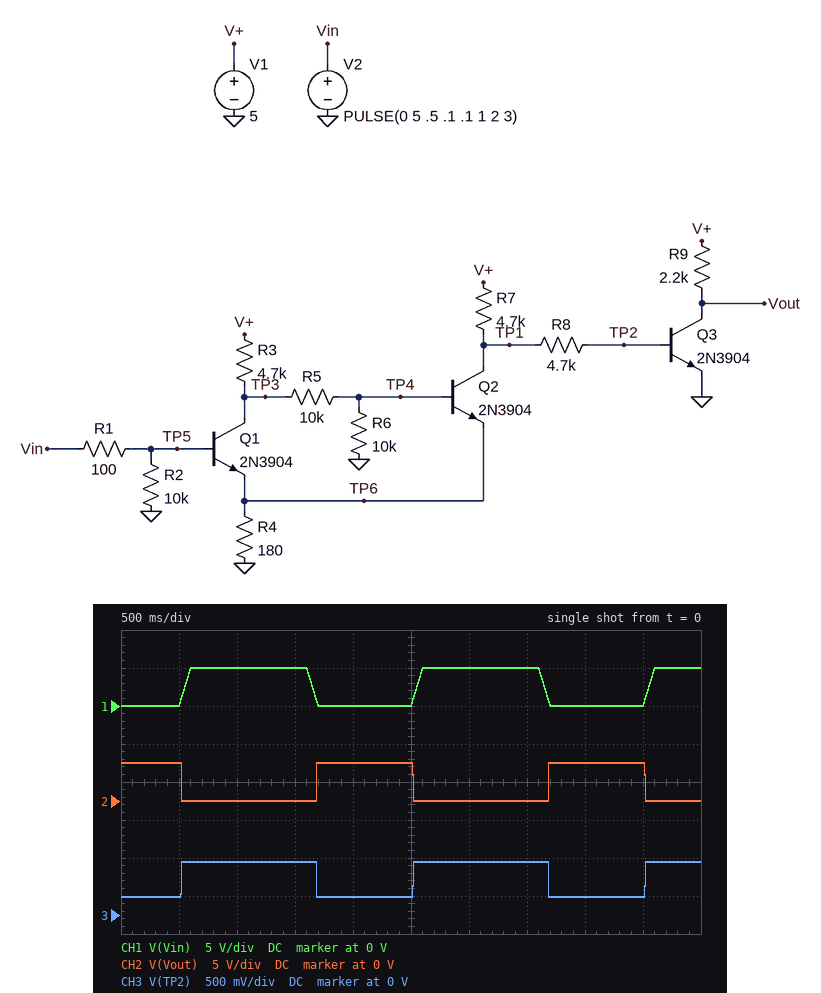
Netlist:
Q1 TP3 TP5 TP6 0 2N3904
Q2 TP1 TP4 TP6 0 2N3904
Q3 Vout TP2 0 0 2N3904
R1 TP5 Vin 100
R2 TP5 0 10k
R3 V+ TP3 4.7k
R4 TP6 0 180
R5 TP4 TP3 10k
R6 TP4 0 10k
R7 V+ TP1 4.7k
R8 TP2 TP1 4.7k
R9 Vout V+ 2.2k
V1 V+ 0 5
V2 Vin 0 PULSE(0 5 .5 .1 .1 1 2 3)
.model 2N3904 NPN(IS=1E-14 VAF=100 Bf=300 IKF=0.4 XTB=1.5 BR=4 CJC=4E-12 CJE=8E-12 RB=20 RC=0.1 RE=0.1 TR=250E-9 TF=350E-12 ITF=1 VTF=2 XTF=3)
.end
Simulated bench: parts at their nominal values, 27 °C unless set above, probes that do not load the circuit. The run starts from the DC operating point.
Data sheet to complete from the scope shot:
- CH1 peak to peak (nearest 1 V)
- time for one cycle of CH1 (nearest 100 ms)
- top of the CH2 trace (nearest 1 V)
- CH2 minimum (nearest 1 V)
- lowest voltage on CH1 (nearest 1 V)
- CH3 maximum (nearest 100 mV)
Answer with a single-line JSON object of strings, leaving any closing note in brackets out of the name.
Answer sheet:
{"CH1 peak to peak": "5 V", "time for one cycle of CH1": "2.0 s", "top of the CH2 trace": "5 V", "CH2 minimum": "0 V", "lowest voltage on CH1": "0 V", "CH3 maximum": "700 mV"}
